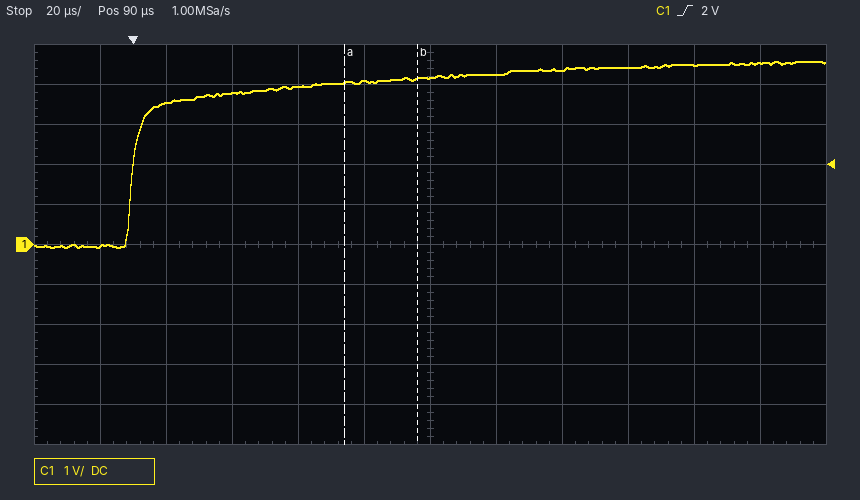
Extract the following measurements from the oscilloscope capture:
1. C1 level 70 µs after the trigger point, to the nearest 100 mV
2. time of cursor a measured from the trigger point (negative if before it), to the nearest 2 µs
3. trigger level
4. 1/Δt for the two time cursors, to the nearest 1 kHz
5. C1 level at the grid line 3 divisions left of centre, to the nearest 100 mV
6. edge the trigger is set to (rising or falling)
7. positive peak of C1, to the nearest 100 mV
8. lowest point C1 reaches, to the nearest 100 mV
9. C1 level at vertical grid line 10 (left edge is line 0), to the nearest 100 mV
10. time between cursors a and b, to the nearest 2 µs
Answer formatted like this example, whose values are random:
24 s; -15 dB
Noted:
4.1 V; +64 µs; 2 V; 45 kHz; 3.8 V; rising; 4.6 V; -100 mV; 4.5 V; 22 µs
